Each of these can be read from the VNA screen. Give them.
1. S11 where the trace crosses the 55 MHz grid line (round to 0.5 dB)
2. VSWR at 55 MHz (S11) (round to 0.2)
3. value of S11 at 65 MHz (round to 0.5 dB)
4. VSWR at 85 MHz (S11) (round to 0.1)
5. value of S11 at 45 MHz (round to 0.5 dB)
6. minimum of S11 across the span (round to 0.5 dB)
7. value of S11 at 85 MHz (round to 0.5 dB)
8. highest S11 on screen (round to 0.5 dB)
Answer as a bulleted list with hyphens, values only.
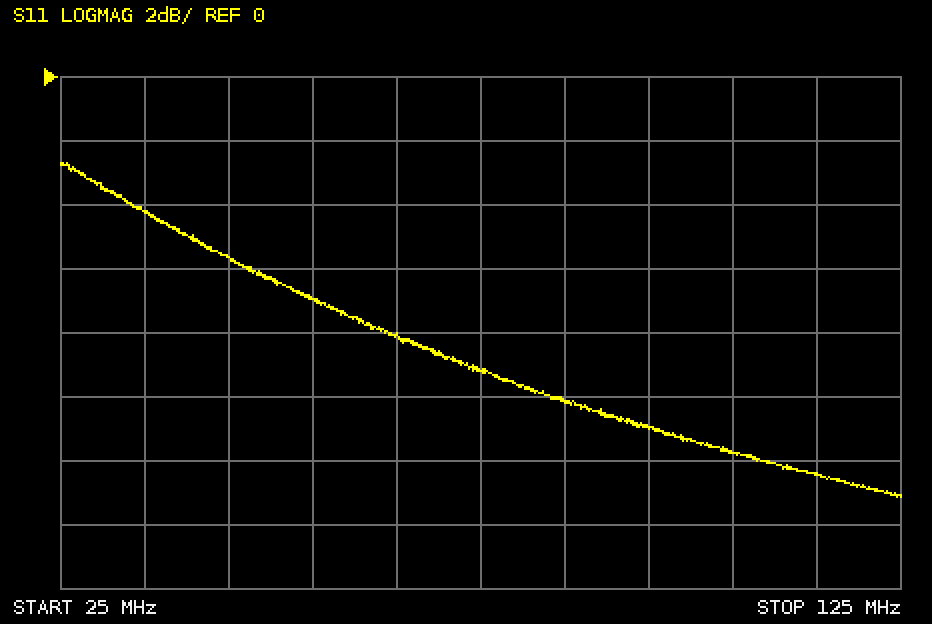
- -7.0 dB
- 2.6
- -8.0 dB
- 1.9
- -5.5 dB
- -13.0 dB
- -10.0 dB
- -2.5 dB
